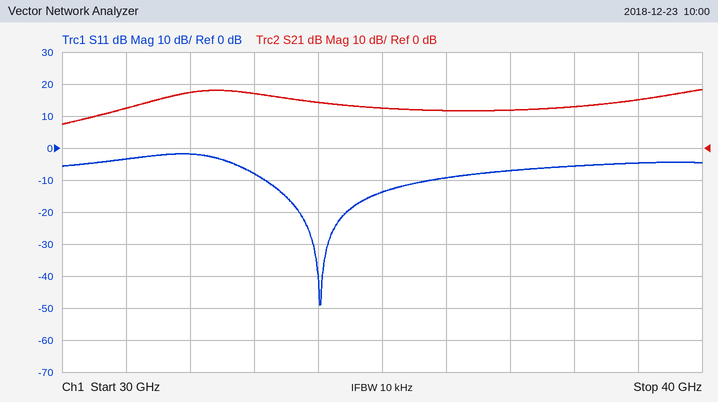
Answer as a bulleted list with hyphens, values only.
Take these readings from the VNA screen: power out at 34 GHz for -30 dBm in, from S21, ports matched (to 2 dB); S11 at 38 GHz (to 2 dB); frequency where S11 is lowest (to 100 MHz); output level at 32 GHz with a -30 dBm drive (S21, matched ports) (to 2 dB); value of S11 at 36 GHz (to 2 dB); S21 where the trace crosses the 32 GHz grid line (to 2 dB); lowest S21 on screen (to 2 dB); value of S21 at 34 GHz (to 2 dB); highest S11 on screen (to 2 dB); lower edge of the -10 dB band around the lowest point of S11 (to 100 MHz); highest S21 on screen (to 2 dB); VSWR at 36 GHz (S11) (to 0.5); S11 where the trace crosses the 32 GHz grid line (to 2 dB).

- -16 dBm
- -6 dB
- 34.0 GHz
- -12 dBm
- -10 dB
- 18 dB
- 8 dB
- 14 dB
- -2 dB
- 33.2 GHz
- 18 dB
- 2.0
- -2 dB
